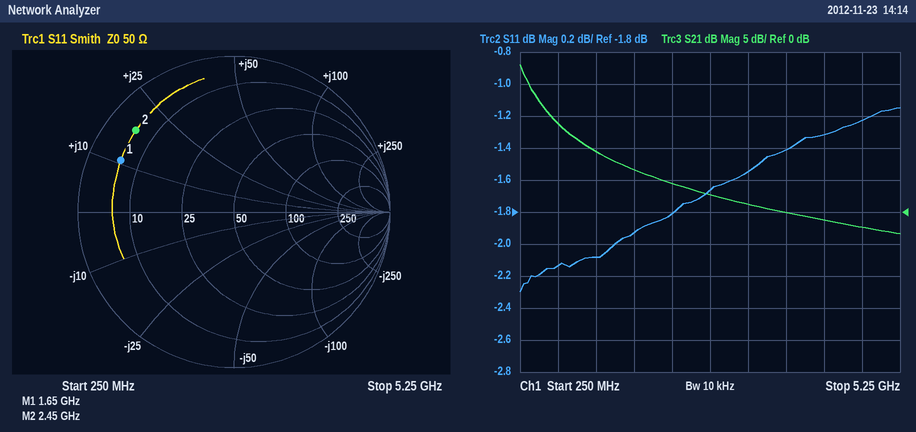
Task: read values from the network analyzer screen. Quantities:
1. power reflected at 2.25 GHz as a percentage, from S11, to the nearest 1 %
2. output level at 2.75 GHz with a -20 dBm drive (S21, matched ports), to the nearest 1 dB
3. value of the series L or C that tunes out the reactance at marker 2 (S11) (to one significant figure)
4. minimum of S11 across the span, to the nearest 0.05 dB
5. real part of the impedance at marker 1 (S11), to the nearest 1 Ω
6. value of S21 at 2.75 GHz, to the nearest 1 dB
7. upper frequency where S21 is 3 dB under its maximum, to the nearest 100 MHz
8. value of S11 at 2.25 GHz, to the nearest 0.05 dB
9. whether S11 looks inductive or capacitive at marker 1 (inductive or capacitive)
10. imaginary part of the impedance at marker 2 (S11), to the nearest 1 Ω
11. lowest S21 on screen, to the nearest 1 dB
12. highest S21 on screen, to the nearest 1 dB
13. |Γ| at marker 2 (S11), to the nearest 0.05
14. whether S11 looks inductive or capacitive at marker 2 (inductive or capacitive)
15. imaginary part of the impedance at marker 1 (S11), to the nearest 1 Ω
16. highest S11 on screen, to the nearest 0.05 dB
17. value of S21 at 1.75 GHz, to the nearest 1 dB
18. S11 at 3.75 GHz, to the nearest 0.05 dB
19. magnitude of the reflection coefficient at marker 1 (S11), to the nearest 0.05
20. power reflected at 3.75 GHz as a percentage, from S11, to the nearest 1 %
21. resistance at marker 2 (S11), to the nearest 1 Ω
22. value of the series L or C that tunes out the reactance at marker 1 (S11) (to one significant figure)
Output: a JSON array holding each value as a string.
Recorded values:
["66 %", "-17 dBm", "4 pF", "-2.30 dB", "6 Ω", "3 dB", "400 MHz", "-1.80 dB", "inductive", "+18 Ω", "-3 dB", "23 dB", "0.80", "inductive", "+11 Ω", "-1.15 dB", "7 dB", "-1.40 dB", "0.80", "72 %", "6 Ω", "9 pF"]
